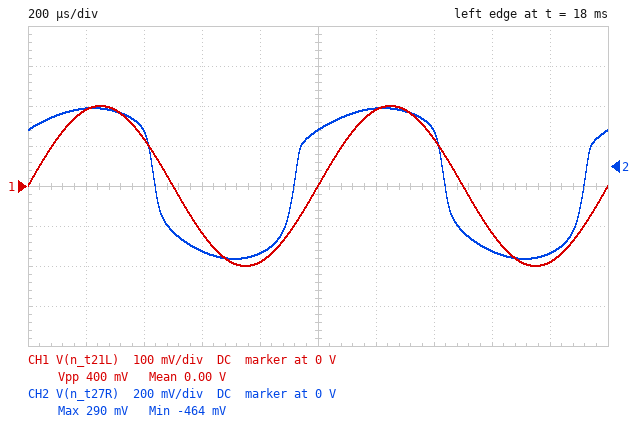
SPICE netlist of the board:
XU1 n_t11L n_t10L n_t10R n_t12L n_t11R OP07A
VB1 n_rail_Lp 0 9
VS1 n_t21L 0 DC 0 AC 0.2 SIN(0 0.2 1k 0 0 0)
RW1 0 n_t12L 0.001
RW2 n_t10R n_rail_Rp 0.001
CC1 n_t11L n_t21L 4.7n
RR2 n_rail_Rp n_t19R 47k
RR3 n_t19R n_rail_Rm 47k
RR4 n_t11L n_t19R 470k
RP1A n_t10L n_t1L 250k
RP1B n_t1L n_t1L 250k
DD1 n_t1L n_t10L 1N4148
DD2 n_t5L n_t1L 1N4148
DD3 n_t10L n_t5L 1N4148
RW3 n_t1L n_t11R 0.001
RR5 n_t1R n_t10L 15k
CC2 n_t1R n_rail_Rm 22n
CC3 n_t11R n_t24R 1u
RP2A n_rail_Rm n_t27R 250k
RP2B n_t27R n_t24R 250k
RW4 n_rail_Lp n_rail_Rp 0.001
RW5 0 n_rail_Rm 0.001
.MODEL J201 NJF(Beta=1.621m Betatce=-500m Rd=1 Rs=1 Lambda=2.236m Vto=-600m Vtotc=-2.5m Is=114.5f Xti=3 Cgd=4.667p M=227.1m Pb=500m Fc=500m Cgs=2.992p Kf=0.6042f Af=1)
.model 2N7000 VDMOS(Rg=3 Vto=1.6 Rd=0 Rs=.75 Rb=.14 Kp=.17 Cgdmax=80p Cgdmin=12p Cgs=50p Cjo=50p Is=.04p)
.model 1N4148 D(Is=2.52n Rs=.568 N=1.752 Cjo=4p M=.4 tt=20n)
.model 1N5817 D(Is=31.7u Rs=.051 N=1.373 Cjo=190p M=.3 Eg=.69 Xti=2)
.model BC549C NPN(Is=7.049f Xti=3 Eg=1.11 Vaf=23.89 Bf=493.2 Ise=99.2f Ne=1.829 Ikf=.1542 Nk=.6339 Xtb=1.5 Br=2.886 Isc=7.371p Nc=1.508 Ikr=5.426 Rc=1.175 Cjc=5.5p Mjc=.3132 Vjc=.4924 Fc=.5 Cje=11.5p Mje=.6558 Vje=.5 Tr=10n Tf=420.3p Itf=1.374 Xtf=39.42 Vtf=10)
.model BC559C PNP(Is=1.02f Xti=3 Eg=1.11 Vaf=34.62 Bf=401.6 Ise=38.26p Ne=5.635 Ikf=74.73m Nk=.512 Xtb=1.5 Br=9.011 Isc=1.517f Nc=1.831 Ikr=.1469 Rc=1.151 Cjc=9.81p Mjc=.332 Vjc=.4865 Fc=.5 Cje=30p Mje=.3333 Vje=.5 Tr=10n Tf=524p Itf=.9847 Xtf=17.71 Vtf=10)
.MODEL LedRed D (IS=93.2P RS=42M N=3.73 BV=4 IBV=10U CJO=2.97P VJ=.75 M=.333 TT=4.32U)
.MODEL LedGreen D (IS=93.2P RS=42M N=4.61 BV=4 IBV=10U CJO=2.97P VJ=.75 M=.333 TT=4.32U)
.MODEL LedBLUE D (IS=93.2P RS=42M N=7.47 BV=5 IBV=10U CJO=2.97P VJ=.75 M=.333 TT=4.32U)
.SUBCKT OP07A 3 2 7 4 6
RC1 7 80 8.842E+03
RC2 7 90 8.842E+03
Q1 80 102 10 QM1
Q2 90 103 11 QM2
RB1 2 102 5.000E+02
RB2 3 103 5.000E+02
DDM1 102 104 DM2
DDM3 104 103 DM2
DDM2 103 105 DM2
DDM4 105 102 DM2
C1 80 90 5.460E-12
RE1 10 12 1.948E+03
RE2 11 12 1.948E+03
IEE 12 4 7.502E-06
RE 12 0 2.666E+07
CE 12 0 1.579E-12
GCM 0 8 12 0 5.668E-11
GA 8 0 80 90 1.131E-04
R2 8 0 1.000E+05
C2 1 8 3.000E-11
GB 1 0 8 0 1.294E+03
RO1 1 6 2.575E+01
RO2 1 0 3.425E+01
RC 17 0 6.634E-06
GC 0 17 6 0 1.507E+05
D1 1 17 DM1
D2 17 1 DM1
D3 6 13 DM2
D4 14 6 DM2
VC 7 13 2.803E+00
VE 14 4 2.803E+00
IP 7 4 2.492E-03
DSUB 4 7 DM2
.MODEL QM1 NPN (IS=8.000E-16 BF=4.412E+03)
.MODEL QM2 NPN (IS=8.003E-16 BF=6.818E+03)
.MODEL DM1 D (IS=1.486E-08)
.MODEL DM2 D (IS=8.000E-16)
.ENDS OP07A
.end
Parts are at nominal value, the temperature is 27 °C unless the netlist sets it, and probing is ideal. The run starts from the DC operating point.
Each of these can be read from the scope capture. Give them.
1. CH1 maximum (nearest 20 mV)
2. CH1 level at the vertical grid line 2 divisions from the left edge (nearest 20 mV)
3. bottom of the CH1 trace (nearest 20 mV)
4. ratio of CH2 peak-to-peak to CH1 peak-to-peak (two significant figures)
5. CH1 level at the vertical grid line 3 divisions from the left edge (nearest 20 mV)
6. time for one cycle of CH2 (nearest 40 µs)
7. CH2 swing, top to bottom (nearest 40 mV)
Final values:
200 mV
120 mV
-200 mV
1.9
-120 mV
1.00 ms
760 mV
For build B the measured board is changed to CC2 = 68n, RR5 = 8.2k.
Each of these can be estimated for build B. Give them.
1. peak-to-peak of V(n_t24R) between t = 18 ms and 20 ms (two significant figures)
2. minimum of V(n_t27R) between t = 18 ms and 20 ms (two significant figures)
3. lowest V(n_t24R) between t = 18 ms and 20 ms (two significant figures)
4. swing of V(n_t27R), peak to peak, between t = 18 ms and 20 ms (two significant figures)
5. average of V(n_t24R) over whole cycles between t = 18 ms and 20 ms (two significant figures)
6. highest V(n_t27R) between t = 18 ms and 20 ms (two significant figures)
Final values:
1.6 V
-500 mV
-1.0 V
810 mV
-170 mV
310 mV
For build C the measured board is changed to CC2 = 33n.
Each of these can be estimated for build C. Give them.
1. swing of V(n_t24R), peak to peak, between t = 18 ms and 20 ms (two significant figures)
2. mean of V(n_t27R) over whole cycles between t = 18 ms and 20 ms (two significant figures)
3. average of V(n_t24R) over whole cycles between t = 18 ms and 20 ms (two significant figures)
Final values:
1.5 V
-73 mV
-150 mV
